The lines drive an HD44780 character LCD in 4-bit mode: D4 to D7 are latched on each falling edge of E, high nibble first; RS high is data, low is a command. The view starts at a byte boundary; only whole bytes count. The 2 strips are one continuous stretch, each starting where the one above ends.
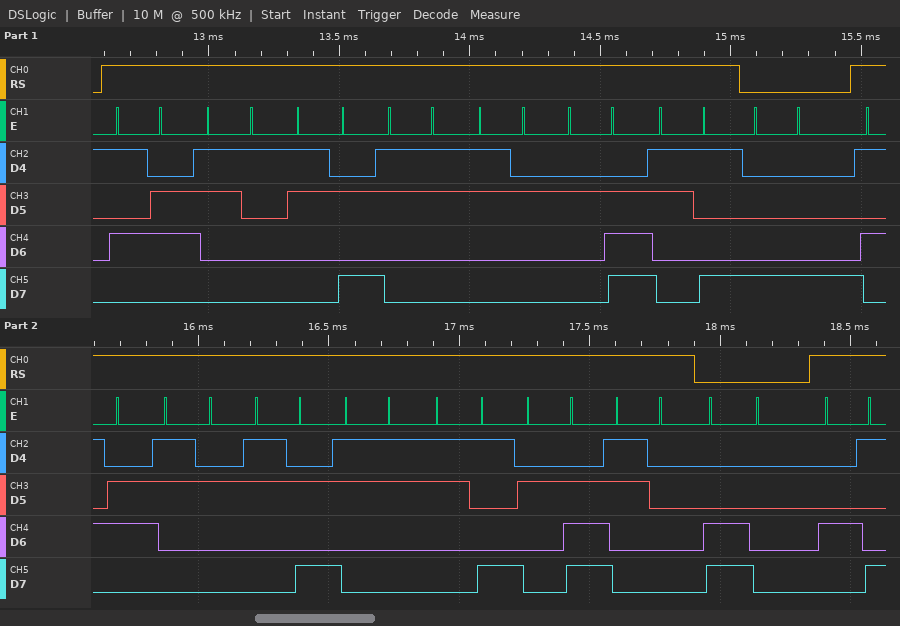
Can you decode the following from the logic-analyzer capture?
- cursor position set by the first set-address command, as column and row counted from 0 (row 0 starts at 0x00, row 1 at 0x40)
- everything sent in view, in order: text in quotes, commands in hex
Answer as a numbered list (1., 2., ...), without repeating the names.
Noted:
1. column 8, row 0
2. "V1:32.9" 0x88 "V2:39.0" 0xC0 "I"
